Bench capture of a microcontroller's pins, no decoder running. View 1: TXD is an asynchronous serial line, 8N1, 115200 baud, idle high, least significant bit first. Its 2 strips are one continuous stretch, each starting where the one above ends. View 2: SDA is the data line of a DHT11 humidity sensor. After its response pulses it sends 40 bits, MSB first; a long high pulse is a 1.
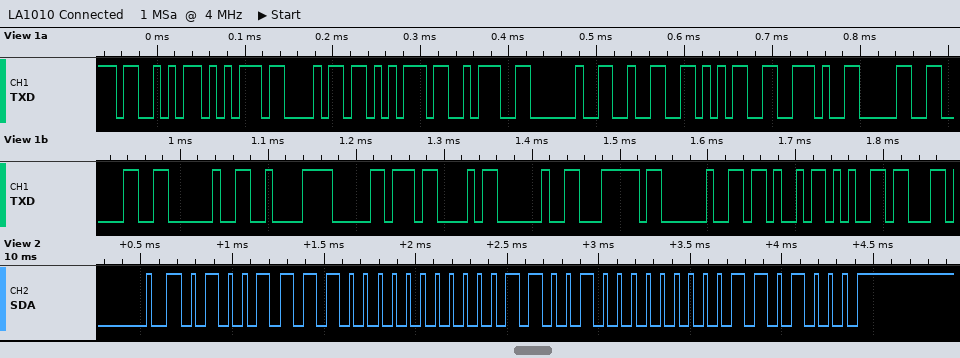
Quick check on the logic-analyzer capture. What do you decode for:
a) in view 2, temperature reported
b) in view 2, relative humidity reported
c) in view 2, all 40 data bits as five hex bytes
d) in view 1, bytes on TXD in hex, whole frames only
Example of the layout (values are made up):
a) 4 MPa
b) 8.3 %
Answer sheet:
a) 25.0 °C
b) 79 %
c) 4F 00 19 00 68
d) 0x53 0x75 0x68 0x75 0x3A 0x20 0x32 0x35 0x2E 0x30 0x30 0x20 0xC2 0xB0 0x43 0x20 0x7C 0x20 0x4B 0x65
